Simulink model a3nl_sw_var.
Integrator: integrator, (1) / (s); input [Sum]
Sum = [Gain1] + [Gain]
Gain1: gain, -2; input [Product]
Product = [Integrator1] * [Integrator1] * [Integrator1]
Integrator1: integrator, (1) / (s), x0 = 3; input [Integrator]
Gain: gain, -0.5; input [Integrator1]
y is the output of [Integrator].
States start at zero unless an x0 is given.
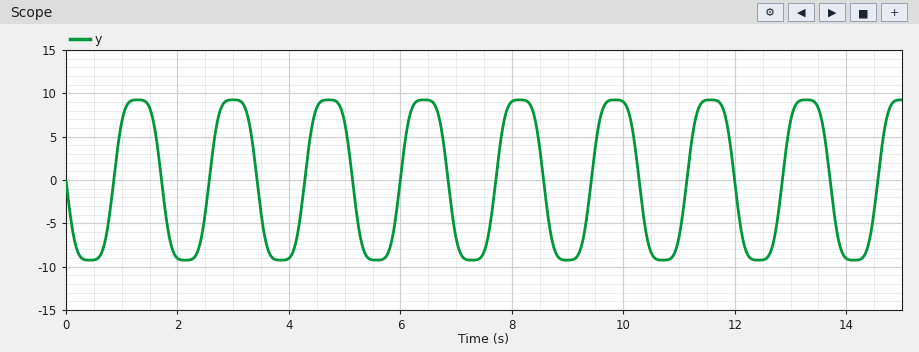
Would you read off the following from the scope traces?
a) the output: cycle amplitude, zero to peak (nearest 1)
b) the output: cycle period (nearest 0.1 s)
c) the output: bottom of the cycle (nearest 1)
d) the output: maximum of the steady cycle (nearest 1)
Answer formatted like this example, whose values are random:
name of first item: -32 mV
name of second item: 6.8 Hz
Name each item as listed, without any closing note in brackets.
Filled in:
the output: cycle amplitude, zero to peak: 9
the output: cycle period: 1.7 s
the output: bottom of the cycle: -9
the output: maximum of the steady cycle: 9
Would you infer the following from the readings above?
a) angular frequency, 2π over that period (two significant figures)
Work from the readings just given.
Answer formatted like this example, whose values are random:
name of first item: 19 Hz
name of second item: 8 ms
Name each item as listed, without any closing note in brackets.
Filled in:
angular frequency, 2π over that period: 3.7 rad/s
